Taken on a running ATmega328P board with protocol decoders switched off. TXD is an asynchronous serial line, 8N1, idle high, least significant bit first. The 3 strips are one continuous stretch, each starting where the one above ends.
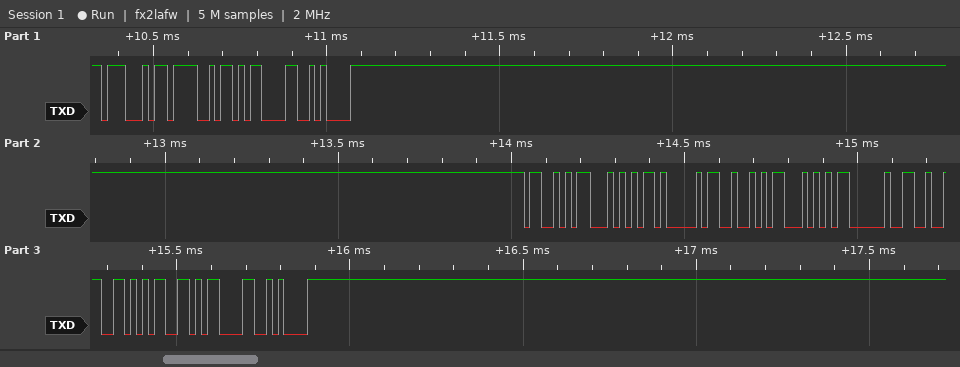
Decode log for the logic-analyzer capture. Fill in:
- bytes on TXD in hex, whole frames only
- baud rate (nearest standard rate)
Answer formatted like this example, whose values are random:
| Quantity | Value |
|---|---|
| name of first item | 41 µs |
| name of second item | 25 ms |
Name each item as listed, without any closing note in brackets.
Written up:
| Quantity | Value |
|---|---|
| bytes on TXD in hex, whole frames only | 0x47 0x4F 0x0D 0x0A 0x53 0x54 0x41 0x52 0x54 0x20 0x32 0x35 0x0D 0x0A |
| baud rate | 57600 baud |
